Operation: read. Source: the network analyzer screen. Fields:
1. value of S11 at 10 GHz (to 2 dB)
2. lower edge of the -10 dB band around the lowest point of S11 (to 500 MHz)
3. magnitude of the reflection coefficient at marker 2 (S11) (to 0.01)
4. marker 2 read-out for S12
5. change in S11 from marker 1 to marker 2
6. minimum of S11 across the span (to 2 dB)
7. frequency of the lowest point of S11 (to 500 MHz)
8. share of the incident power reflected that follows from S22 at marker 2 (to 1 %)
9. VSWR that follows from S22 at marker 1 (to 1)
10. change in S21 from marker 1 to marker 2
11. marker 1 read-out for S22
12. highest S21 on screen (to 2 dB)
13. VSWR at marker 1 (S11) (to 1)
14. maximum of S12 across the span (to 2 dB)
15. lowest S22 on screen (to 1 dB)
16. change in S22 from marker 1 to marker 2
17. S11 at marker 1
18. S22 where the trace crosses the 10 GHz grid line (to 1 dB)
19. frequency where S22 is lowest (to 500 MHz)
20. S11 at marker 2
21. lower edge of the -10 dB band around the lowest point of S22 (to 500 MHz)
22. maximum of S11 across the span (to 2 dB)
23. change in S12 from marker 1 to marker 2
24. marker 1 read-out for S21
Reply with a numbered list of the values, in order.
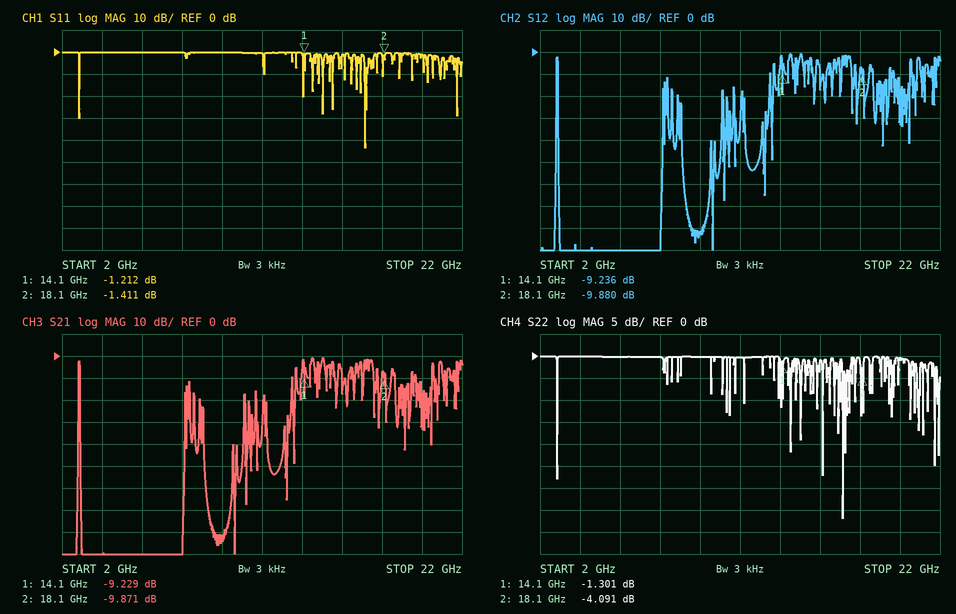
1. 0 dB
2. 17.0 GHz
3. 0.85
4. -9.880 dB
5. -0.199 dB
6. -44 dB
7. 17.0 GHz
8. 39 %
9. 13
10. -0.642 dB
11. -1.301 dB
12. 0 dB
13. 14
14. 0 dB
15. -37 dB
16. -2.790 dB
17. -1.212 dB
18. 0 dB
19. 17.0 GHz
20. -1.411 dB
21. 17.0 GHz
22. 0 dB
23. -0.644 dB
24. -9.229 dB
